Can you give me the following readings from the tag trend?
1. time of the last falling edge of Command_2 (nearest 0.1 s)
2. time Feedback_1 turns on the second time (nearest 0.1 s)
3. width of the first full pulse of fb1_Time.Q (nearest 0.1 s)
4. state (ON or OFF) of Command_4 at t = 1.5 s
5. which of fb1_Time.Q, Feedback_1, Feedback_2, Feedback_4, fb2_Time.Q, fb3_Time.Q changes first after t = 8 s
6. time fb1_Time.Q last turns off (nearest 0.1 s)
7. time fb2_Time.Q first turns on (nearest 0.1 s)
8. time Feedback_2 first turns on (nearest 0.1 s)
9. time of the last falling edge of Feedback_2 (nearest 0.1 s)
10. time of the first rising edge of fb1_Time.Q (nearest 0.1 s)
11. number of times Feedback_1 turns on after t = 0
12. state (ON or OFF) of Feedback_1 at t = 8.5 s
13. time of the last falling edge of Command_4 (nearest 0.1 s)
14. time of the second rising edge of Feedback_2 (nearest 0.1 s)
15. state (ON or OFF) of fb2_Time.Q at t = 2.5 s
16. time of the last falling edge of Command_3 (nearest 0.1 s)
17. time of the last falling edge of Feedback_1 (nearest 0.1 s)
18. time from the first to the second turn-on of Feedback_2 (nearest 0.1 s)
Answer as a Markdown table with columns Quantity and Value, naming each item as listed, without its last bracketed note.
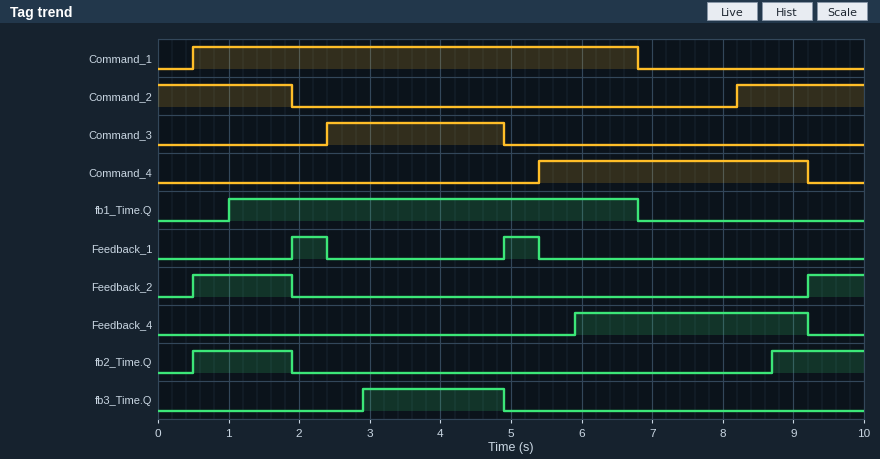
| Quantity | Value |
|---|---|
| time of the last falling edge of Command_2 | 1.9 s |
| time Feedback_1 turns on the second time | 4.9 s |
| width of the first full pulse of fb1_Time.Q | 5.8 s |
| state (ON or OFF) of Command_4 at t = 1.5 s | OFF |
| which of fb1_Time.Q, Feedback_1, Feedback_2, Feedback_4, fb2_Time.Q, fb3_Time.Q changes first after t = 8 s | fb2_Time.Q |
| time fb1_Time.Q last turns off | 6.8 s |
| time fb2_Time.Q first turns on | 0.5 s |
| time Feedback_2 first turns on | 0.5 s |
| time of the last falling edge of Feedback_2 | 1.9 s |
| time of the first rising edge of fb1_Time.Q | 1.0 s |
| number of times Feedback_1 turns on after t = 0 | 2 |
| state (ON or OFF) of Feedback_1 at t = 8.5 s | OFF |
| time of the last falling edge of Command_4 | 9.2 s |
| time of the second rising edge of Feedback_2 | 9.2 s |
| state (ON or OFF) of fb2_Time.Q at t = 2.5 s | OFF |
| time of the last falling edge of Command_3 | 4.9 s |
| time of the last falling edge of Feedback_1 | 5.4 s |
| time from the first to the second turn-on of Feedback_2 | 8.7 s |
